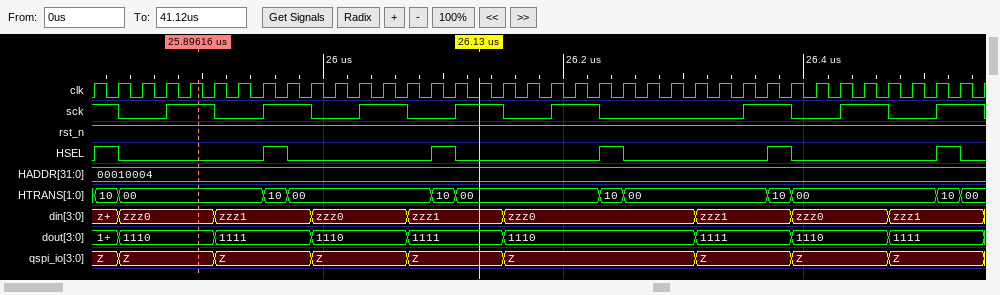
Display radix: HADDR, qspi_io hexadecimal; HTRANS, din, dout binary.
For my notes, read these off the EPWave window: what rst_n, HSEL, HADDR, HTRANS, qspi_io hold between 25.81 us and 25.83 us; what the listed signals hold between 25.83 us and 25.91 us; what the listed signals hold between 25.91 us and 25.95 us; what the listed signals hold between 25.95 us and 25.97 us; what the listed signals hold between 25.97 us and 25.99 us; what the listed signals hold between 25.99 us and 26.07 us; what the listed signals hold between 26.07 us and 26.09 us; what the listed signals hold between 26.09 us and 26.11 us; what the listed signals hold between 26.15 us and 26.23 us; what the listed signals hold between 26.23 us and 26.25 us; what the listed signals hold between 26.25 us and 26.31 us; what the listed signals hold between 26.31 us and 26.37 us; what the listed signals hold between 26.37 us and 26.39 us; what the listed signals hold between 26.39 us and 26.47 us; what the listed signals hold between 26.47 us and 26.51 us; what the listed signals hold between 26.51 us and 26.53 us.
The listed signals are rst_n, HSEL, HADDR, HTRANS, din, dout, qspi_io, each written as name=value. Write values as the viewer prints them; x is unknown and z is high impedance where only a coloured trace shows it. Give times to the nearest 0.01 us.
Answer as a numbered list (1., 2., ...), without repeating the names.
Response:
1. rst_n=1, HSEL=1, HADDR=00010004, HTRANS=10, qspi_io=Z
2. rst_n=1, HSEL=0, HADDR=00010004, HTRANS=00, din=zzz0, dout=1110, qspi_io=Z
3. rst_n=1, HSEL=0, HADDR=00010004, HTRANS=00, din=zzz1, dout=1111, qspi_io=Z
4. rst_n=1, HSEL=1, HADDR=00010004, HTRANS=10, din=zzz1, dout=1111, qspi_io=Z
5. rst_n=1, HSEL=0, HADDR=00010004, HTRANS=00, din=zzz1, dout=1111, qspi_io=Z
6. rst_n=1, HSEL=0, HADDR=00010004, HTRANS=00, din=zzz0, dout=1110, qspi_io=Z
7. rst_n=1, HSEL=0, HADDR=00010004, HTRANS=00, din=zzz1, dout=1111, qspi_io=Z
8. rst_n=1, HSEL=1, HADDR=00010004, HTRANS=10, din=zzz1, dout=1111, qspi_io=Z
9. rst_n=1, HSEL=0, HADDR=00010004, HTRANS=00, din=zzz0, dout=1110, qspi_io=Z
10. rst_n=1, HSEL=1, HADDR=00010004, HTRANS=10, din=zzz0, dout=1110, qspi_io=Z
11. rst_n=1, HSEL=0, HADDR=00010004, HTRANS=00, din=zzz0, dout=1110, qspi_io=Z
12. rst_n=1, HSEL=0, HADDR=00010004, HTRANS=00, din=zzz1, dout=1111, qspi_io=Z
13. rst_n=1, HSEL=1, HADDR=00010004, HTRANS=10, din=zzz1, dout=1111, qspi_io=Z
14. rst_n=1, HSEL=0, HADDR=00010004, HTRANS=00, din=zzz0, dout=1110, qspi_io=Z
15. rst_n=1, HSEL=0, HADDR=00010004, HTRANS=00, din=zzz1, dout=1111, qspi_io=Z
16. rst_n=1, HSEL=1, HADDR=00010004, HTRANS=10, din=zzz1, dout=1111, qspi_io=Z
